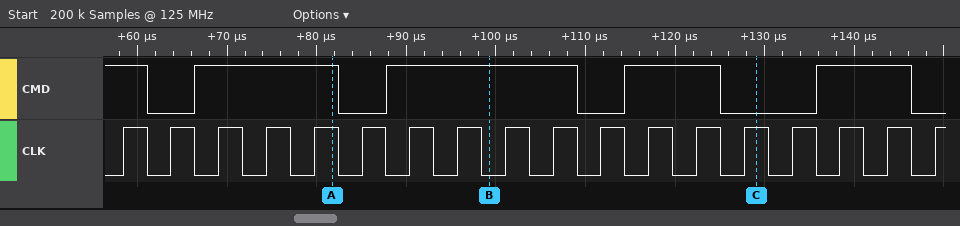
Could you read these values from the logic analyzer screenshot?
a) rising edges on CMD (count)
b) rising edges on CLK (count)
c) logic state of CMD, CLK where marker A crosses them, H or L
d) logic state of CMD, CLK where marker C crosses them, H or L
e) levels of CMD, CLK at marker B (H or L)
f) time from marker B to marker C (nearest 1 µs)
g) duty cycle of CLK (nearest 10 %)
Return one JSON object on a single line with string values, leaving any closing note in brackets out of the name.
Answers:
{"rising edges on CMD": "4", "rising edges on CLK": "18", "logic state of CMD, CLK where marker A crosses them, H or L": "CMD=H, CLK=H", "logic state of CMD, CLK where marker C crosses them, H or L": "CMD=L, CLK=H", "levels of CMD, CLK at marker B": "CMD=H, CLK=L", "time from marker B to marker C": "30 µs", "duty cycle of CLK": "50 %"}
